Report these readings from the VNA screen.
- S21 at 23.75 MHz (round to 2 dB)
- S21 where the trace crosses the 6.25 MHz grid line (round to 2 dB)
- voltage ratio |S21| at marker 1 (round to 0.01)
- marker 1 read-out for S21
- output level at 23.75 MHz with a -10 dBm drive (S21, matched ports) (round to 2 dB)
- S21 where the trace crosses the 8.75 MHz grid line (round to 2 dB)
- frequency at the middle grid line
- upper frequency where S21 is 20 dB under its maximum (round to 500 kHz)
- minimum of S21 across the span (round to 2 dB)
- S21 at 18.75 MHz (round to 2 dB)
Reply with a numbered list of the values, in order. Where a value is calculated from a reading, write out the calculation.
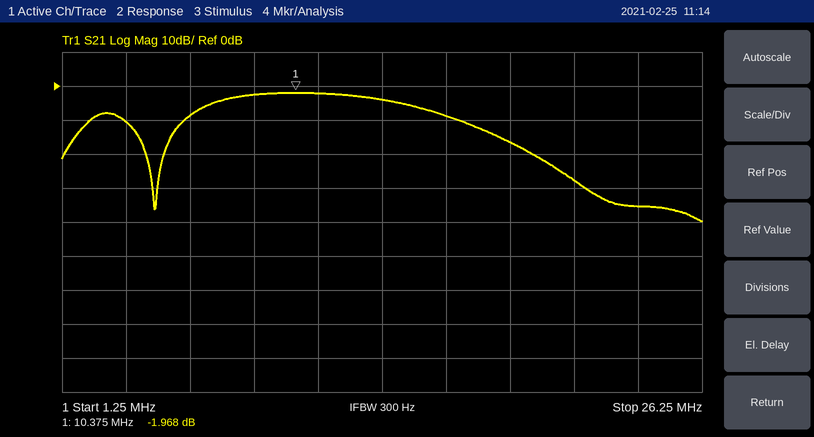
1. -36 dB
2. -8 dB
3. 10^(-1.968/20) ≈ 0.80
4. -1.968 dB
5. -10 dBm + (-36 dB) = -46 dBm
6. -2 dB
7. 13.75 MHz
8. 20.0 MHz
9. -40 dB
10. -16 dB
